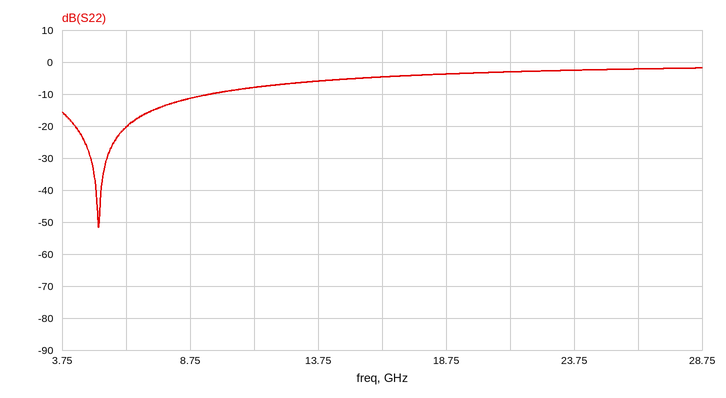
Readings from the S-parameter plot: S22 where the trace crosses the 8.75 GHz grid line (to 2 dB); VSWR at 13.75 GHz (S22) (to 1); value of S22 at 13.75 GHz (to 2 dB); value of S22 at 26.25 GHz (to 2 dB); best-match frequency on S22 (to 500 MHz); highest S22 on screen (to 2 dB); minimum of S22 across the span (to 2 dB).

-12 dB
3
-6 dB
-2 dB
5.0 GHz
-2 dB
-52 dB
